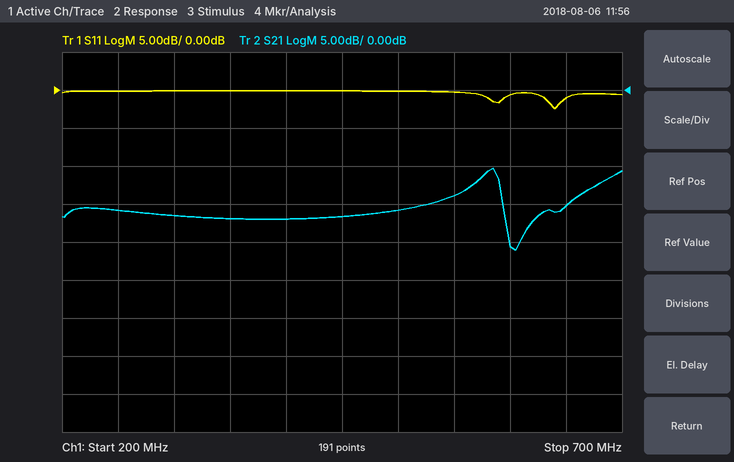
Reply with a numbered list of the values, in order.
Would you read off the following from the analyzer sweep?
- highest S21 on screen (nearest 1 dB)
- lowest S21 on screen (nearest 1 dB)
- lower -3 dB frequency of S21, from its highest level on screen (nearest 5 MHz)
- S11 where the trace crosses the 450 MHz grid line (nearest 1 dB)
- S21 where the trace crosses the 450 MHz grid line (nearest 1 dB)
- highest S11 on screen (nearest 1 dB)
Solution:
1. -10 dB
2. -21 dB
3. 560 MHz
4. 0 dB
5. -17 dB
6. 0 dB
